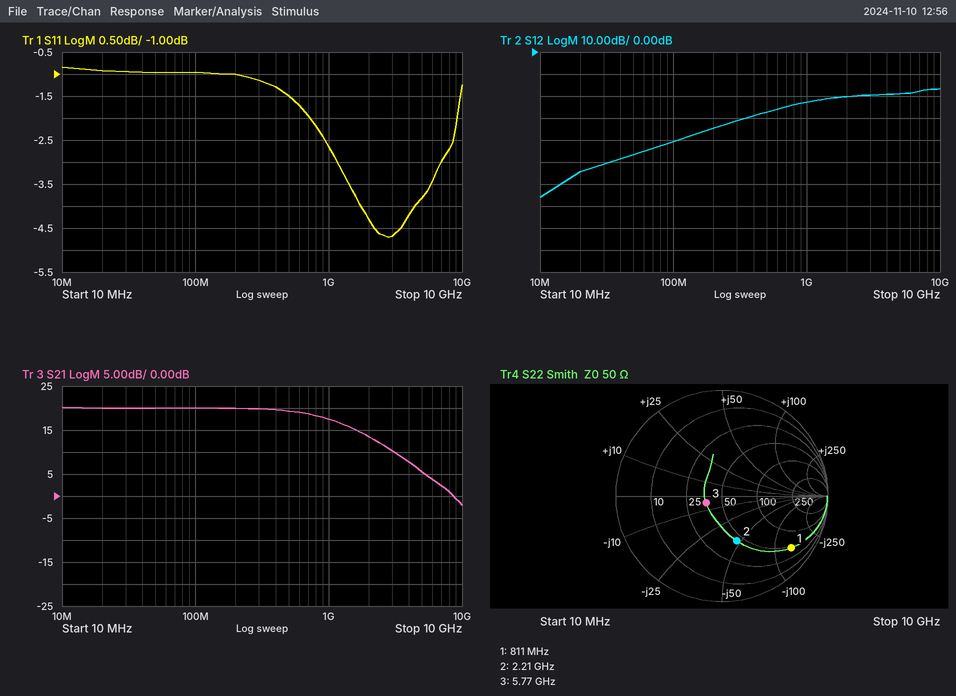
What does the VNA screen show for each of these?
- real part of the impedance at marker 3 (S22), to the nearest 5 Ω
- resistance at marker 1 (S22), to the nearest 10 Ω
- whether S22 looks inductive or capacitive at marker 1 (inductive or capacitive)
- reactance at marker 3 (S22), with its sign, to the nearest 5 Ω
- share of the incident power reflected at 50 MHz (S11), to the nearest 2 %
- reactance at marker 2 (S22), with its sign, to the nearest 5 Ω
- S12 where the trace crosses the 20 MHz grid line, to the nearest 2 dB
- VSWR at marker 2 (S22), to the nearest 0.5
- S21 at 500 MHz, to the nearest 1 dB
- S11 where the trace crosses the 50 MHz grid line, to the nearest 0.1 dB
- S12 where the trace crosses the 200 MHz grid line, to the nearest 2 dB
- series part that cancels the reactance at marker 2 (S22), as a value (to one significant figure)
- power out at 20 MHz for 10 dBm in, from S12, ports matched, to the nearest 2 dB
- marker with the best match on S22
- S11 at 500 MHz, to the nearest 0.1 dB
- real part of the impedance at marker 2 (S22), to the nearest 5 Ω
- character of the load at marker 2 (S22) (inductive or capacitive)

35 Ω
50 Ω
capacitive
-5 Ω
80 %
-45 Ω
-54 dB
2.5
19 dB
-1.0 dB
-34 dB
3 nH
-44 dBm
marker 3
-1.5 dB
45 Ω
capacitive
